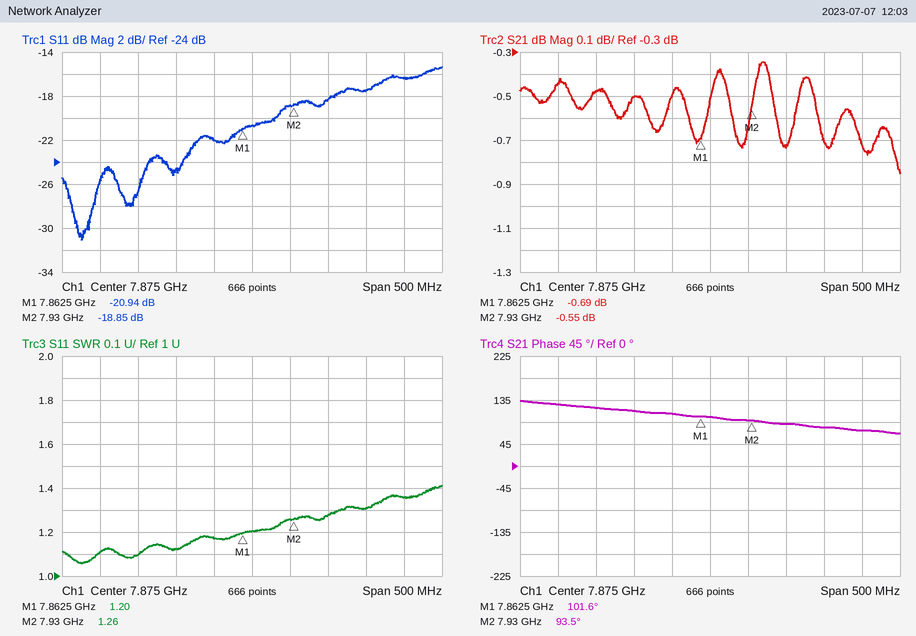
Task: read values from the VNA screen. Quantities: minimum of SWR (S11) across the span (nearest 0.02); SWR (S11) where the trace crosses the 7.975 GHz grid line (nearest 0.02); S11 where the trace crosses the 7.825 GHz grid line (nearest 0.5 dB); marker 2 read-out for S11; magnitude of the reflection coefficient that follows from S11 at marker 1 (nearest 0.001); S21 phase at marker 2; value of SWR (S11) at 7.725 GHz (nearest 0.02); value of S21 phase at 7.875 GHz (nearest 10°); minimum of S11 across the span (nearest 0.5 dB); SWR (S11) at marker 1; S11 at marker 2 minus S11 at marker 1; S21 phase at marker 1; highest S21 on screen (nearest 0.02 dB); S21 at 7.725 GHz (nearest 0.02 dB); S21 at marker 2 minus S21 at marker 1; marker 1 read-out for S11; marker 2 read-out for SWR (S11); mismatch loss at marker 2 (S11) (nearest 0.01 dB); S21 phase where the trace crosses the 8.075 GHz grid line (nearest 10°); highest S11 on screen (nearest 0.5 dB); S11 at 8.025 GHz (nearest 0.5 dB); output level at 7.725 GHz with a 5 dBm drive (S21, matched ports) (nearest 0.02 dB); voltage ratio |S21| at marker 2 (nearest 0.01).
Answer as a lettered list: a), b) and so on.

a) 1.06
b) 1.28
c) -22.0 dB
d) -18.85 dB
e) 0.090
f) 93.5°
g) 1.10
h) 100°
i) -31.0 dB
j) 1.20
k) 2.09 dB
l) 101.6°
m) -0.34 dB
n) -0.48 dB
o) 0.14 dB
p) -20.94 dB
q) 1.26
r) 0.06 dB
s) 70°
t) -15.5 dB
u) -17.5 dB
v) 4.52 dBm
w) 0.94
